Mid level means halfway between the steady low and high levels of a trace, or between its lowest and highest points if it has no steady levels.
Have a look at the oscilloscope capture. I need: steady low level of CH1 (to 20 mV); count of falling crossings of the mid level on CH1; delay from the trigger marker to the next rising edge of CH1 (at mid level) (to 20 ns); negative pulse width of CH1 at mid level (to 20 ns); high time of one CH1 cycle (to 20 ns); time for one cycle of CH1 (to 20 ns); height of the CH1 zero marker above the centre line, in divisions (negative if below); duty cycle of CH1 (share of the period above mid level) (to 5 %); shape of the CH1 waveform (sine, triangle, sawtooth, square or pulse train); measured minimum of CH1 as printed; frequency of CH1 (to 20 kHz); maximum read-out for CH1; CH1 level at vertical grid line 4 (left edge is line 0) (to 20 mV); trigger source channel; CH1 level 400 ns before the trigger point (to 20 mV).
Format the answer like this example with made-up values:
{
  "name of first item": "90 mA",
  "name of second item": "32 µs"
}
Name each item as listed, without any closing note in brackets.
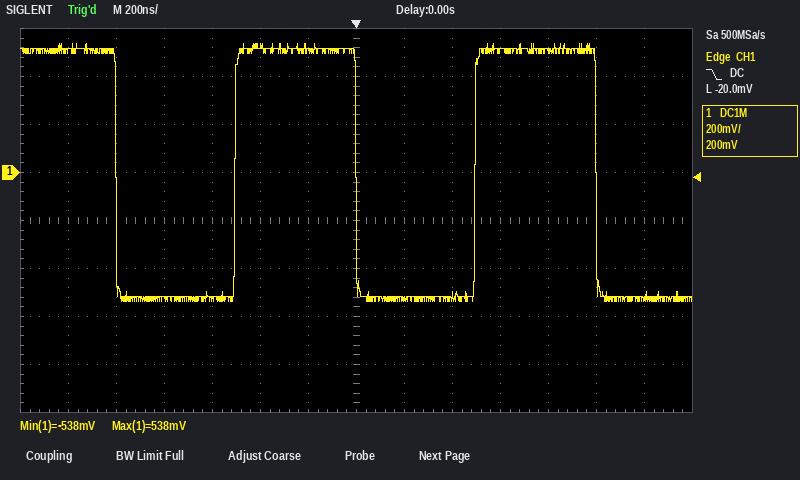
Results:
{
  "steady low level of CH1": "-520 mV",
  "count of falling crossings of the mid level on CH1": "3",
  "delay from the trigger marker to the next rising edge of CH1 (at mid level)": "500 ns",
  "negative pulse width of CH1 at mid level": "500 ns",
  "high time of one CH1 cycle": "500 ns",
  "time for one cycle of CH1": "1.00 µs",
  "height of the CH1 zero marker above the centre line, in divisions": "+1.0 div",
  "duty cycle of CH1 (share of the period above mid level)": "50 %",
  "shape of the CH1 waveform": "square",
  "measured minimum of CH1 as printed": "-538 mV",
  "frequency of CH1": "1.00 MHz",
  "maximum read-out for CH1": "538 mV",
  "CH1 level at vertical grid line 4 (left edge is line 0)": "-520 mV",
  "trigger source channel": "CH1",
  "CH1 level 400 ns before the trigger point": "520 mV"
}
